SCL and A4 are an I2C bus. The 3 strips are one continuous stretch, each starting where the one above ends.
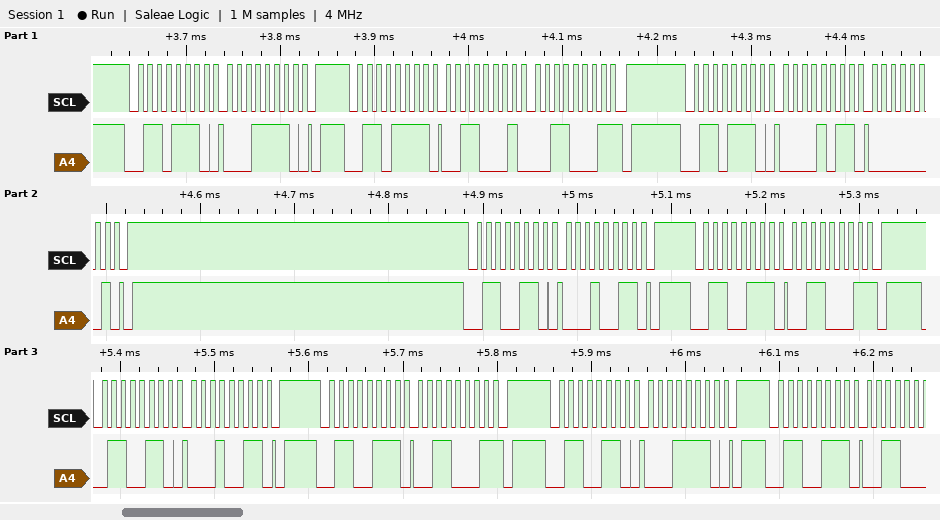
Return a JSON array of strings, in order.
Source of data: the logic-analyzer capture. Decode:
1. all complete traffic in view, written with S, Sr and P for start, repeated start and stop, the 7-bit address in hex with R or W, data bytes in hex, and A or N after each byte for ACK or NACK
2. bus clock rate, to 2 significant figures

["S 37W A 1E A P S 37R A 31 A 31 N P S 37W A 0B A 01 A P S 33W A 13 A P S 33R A 31 N P S 33W A 13 A P S 33R A 31 N P S 33W A 1E A P S 33R A", "100 kHz"]
